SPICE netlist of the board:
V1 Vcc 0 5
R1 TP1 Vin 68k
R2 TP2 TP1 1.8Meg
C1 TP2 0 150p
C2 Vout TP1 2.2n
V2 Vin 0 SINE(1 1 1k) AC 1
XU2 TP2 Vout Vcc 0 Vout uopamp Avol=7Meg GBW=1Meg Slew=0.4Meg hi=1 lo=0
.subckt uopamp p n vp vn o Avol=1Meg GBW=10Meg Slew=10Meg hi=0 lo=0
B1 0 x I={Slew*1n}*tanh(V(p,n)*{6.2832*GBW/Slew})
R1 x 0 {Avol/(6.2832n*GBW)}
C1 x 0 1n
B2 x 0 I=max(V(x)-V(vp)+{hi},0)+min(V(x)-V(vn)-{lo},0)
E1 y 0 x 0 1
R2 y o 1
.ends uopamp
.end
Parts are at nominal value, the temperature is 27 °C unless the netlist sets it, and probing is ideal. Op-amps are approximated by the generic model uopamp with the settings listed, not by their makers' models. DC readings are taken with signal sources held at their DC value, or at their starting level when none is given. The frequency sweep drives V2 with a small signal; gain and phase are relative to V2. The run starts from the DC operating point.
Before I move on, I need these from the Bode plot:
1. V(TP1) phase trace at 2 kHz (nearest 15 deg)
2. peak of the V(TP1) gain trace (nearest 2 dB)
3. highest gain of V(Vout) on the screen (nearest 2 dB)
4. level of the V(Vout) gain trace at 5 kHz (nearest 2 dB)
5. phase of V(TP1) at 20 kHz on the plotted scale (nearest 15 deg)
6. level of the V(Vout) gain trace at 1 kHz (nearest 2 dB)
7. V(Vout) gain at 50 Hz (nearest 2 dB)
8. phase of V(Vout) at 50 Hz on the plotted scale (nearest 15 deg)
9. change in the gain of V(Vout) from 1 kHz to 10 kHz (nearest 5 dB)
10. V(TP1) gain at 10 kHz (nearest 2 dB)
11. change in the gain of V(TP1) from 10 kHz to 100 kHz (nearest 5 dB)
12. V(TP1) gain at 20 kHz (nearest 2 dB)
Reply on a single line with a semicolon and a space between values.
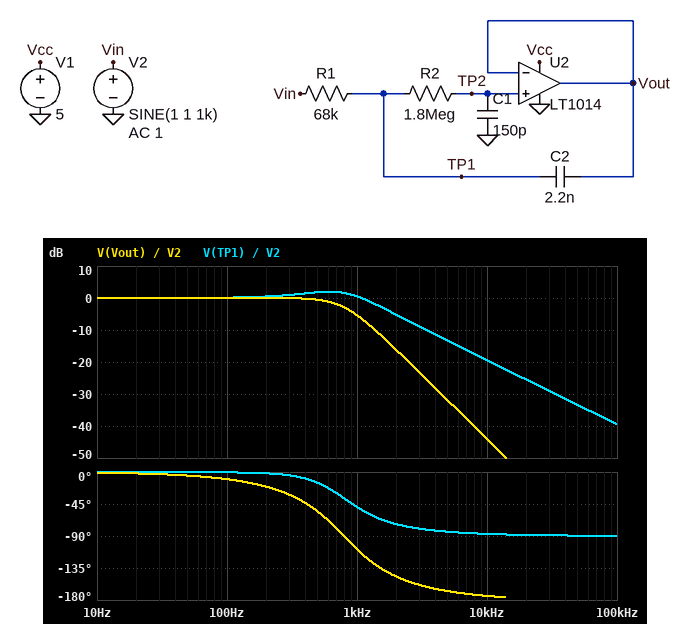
-75 deg; 2 dB; 0 dB; -32 dB; -90 deg; -6 dB; 0 dB; 0 deg; -40 dB; -20 dB; -20 dB; -26 dB
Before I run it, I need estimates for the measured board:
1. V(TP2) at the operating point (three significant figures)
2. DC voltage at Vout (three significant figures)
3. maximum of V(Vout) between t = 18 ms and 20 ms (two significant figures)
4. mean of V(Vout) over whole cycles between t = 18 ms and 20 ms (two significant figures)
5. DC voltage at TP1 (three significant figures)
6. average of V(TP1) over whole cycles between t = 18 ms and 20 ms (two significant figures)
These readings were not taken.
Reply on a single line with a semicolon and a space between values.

1.00 V; 1.00 V; 1.5 V; 1.0 V; 1.00 V; 1.0 V
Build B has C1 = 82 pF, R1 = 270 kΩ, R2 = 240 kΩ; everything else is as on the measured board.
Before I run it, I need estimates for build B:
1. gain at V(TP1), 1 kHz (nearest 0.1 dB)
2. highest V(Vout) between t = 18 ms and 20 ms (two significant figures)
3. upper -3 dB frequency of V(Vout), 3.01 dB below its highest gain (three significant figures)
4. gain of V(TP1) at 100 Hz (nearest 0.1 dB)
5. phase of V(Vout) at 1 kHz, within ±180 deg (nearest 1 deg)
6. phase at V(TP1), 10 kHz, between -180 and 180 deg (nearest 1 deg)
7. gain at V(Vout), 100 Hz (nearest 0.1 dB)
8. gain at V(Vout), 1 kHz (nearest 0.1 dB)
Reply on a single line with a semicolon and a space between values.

4.6 dB; 2.9 V; 1.67 kHz; 0 dB; -26 deg; -126 deg; 0 dB; 4.5 dB
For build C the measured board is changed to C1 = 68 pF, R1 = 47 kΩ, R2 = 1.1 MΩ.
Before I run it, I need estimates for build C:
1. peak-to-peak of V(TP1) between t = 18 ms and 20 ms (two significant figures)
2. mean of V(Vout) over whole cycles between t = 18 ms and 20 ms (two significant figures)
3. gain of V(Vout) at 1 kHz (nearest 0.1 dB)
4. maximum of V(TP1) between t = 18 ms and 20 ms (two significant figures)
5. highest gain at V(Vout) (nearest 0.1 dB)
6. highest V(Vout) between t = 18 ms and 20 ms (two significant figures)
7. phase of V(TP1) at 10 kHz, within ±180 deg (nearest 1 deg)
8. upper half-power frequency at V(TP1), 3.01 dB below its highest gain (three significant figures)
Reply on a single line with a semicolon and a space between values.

2.6 V; 1.0 V; 1.4 dB; 2.3 V; 2.0 dB; 2.2 V; -93 deg; 2.38 kHz
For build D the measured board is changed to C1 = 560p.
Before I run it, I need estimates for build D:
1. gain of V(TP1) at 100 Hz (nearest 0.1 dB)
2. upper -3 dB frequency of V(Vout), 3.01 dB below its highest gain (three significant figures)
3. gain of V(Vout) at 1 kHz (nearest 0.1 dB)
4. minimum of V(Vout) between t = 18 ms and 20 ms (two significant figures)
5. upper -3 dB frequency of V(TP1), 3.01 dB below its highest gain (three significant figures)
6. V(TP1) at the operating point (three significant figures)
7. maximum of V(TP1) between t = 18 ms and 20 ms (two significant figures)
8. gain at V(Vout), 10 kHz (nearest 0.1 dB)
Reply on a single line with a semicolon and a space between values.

0.3 dB; 176 Hz; -18.3 dB; 880 mV; 1.06 kHz; 1.00 V; 1.8 V; -55.5 dB
